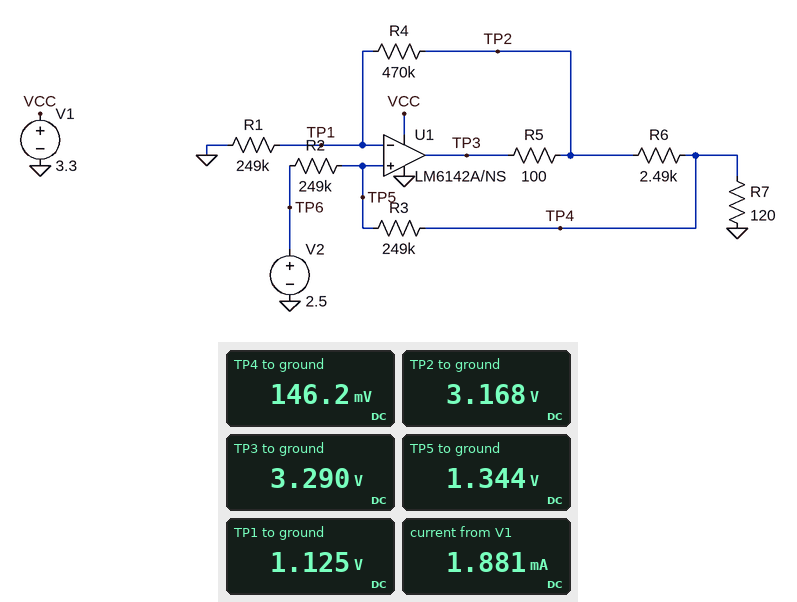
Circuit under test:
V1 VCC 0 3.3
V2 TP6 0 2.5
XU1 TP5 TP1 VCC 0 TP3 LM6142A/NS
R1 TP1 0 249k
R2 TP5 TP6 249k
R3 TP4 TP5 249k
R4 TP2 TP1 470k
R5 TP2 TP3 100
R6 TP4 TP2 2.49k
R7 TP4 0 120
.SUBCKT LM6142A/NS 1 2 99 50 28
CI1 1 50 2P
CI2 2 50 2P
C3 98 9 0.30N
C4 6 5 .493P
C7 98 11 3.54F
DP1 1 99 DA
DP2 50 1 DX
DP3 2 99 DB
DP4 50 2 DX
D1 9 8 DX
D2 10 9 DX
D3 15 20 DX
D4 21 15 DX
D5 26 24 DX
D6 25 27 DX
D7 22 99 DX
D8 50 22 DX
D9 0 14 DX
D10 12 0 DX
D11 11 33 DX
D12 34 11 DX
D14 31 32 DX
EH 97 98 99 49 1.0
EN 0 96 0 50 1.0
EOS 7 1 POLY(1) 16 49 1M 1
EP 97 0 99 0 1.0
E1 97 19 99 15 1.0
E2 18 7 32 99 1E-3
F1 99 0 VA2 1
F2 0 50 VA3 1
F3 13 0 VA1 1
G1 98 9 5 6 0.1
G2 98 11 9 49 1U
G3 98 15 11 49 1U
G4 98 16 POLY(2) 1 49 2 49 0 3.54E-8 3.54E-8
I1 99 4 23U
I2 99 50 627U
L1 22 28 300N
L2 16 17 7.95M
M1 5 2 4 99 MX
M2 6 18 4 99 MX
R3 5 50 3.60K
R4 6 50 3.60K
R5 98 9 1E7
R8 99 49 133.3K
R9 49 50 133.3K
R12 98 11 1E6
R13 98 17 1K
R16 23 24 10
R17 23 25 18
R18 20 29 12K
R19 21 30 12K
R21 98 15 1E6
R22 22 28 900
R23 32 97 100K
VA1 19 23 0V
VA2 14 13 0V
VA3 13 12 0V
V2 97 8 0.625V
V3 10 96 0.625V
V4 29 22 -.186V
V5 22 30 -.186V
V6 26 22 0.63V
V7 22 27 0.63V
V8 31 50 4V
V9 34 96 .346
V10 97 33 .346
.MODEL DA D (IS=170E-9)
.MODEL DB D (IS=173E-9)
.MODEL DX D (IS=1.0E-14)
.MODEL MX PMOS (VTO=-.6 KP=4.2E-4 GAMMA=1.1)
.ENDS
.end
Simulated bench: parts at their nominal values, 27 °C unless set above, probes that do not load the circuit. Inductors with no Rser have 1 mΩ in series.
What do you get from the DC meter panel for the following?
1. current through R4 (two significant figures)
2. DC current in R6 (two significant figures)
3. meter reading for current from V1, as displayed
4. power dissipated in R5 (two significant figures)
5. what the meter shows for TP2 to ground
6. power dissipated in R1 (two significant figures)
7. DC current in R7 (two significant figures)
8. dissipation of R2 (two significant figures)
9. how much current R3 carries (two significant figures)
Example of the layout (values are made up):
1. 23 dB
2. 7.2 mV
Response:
1. 4.3 µA
2. 1.2 mA
3. 1.881 mA
4. 150 µW
5. 3.168 V
6. 5.1 µW
7. 1.2 mA
8. 5.4 µW
9. 4.8 µA
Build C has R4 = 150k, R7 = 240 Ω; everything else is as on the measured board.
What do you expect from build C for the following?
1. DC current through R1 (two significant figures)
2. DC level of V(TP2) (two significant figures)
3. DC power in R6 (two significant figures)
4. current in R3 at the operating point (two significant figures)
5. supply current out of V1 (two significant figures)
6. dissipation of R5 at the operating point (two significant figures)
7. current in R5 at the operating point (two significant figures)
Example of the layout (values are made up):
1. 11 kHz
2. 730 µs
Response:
1. 5.5 µA
2. 2.2 V
3. 1.6 mW
4. 4.7 µA
5. 1.5 mA
6. 64 µW
7. 800 µA
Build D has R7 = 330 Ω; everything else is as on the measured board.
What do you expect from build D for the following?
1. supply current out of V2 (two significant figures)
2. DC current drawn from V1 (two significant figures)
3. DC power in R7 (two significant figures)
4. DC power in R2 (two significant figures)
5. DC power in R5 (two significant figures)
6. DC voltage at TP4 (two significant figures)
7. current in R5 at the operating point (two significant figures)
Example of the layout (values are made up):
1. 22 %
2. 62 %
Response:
1. 4.2 µA
2. 1.8 mA
3. 420 µW
4. 4.4 µW
5. 130 µW
6. 370 mV
7. 1.1 mA
